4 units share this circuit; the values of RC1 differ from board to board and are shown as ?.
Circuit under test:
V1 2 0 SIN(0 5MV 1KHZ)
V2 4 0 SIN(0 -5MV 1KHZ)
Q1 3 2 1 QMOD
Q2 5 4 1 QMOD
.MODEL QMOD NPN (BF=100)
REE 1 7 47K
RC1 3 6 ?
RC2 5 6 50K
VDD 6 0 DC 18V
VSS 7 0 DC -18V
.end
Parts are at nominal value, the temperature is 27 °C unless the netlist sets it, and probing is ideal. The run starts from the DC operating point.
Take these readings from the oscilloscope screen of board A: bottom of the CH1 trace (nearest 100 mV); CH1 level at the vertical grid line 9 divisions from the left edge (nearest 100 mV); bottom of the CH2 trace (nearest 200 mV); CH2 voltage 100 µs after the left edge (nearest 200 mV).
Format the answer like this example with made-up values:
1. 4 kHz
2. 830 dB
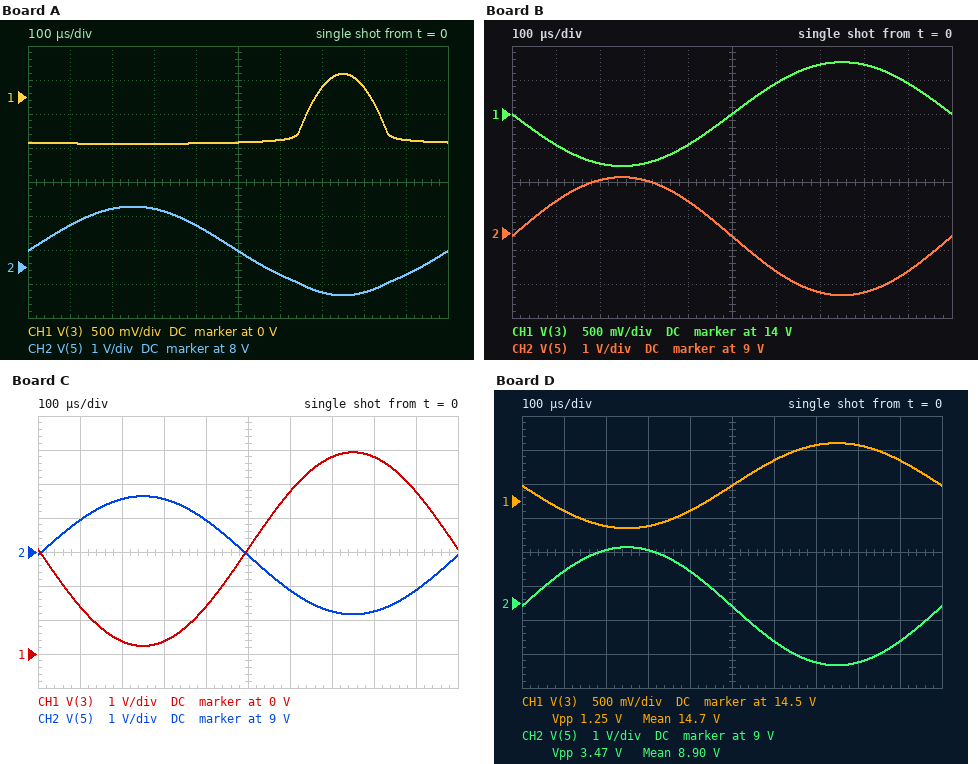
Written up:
1. -700 mV
2. -600 mV
3. 7.2 V
4. 9.2 V
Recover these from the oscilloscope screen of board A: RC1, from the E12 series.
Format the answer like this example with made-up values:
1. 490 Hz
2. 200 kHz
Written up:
1. 120 kΩ
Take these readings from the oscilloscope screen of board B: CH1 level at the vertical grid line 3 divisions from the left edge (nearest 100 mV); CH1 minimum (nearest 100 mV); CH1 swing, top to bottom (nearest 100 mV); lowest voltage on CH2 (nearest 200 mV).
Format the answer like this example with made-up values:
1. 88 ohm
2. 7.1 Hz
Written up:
1. 13.3 V
2. 13.2 V
3. 1.5 V
4. 7.2 V
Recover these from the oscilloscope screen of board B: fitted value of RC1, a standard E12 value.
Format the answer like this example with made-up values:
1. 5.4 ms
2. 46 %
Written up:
1. 22 kΩ
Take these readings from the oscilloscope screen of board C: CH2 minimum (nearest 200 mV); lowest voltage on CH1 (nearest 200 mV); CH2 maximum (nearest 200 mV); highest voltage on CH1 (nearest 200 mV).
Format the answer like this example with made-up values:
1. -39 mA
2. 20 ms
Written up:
1. 7.2 V
2. 200 mV
3. 10.6 V
4. 6.0 V
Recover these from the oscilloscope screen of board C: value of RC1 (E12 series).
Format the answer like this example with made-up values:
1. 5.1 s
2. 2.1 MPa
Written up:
1. 82 kΩ
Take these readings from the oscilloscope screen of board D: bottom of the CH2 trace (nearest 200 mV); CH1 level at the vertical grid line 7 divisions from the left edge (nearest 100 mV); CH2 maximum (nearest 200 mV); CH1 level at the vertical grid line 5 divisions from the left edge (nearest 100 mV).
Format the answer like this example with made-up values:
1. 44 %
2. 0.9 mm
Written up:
1. 7.2 V
2. 15.3 V
3. 10.6 V
4. 14.7 V
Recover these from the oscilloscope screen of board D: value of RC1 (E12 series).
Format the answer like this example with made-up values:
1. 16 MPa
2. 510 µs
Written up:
1. 18 kΩ
